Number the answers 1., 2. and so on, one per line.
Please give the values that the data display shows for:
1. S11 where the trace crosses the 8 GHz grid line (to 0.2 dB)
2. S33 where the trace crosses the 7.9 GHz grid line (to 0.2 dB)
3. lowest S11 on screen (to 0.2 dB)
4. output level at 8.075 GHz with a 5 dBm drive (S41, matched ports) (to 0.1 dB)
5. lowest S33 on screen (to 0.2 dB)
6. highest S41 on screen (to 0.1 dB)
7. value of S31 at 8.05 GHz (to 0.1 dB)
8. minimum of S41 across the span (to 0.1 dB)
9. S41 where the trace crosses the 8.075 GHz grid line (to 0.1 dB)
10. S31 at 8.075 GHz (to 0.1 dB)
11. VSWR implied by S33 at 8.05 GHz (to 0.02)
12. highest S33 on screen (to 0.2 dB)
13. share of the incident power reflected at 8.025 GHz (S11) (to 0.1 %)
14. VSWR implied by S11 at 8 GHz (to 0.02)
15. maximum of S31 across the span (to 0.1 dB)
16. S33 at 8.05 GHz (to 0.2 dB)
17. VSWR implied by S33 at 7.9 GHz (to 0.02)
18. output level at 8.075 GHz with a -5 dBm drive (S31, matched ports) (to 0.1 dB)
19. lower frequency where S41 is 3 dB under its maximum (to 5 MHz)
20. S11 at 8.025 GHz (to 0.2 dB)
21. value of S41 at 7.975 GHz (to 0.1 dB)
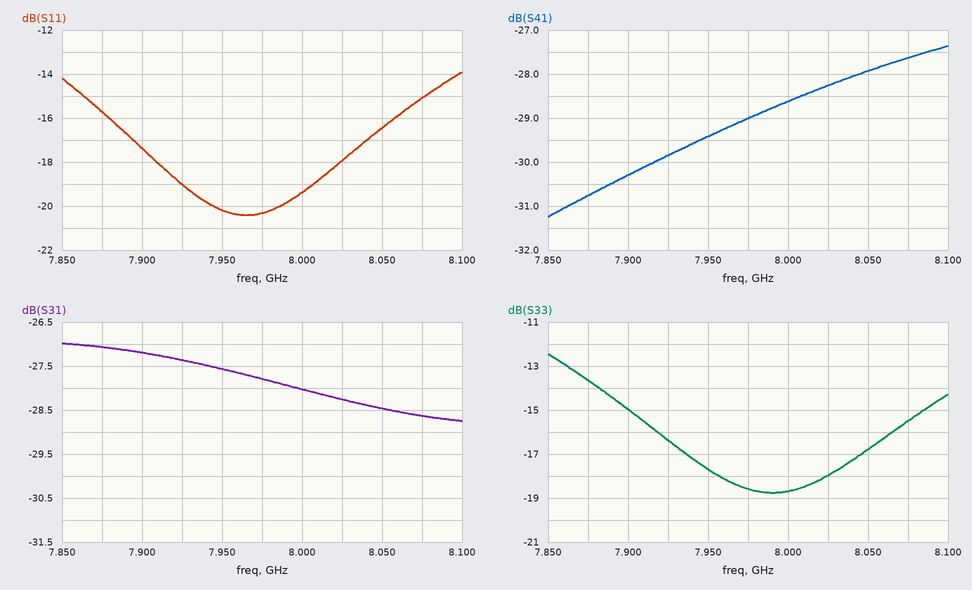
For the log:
1. -19.4 dB
2. -15.0 dB
3. -20.4 dB
4. -22.6 dBm
5. -18.8 dB
6. -27.4 dB
7. -28.5 dB
8. -31.2 dB
9. -27.6 dB
10. -28.6 dB
11. 1.34
12. -12.4 dB
13. 1.6 %
14. 1.24
15. -27.0 dB
16. -16.8 dB
17. 1.44
18. -33.6 dBm
19. 7.895 GHz
20. -18.0 dB
21. -29.0 dB
